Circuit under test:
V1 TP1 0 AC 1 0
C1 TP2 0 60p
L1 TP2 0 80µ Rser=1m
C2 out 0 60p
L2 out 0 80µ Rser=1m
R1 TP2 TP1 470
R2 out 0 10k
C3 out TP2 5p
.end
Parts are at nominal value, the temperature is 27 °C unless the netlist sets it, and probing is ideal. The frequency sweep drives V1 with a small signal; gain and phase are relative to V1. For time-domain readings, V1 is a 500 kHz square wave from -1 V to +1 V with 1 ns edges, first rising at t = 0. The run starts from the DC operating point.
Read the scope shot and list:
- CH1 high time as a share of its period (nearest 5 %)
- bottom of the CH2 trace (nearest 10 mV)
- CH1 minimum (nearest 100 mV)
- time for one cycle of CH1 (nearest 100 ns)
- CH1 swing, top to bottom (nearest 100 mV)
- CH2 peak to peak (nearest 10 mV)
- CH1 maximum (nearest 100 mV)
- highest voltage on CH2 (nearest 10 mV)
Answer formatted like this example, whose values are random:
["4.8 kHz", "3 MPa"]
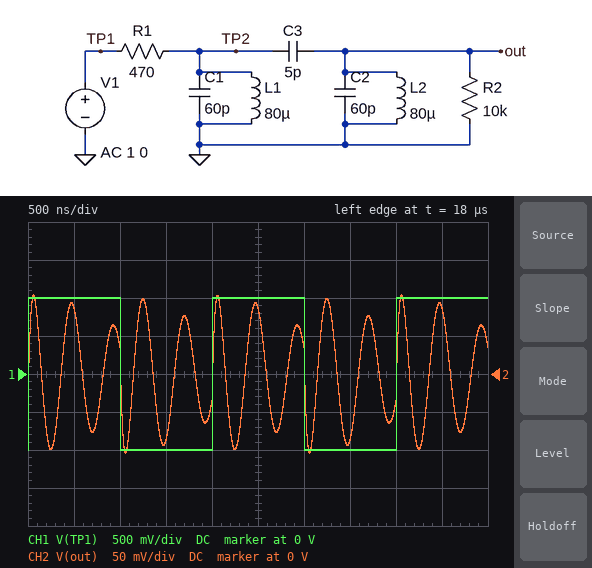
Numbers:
["50 %", "-100 mV", "-1.0 V", "2.0 µs", "2.0 V", "210 mV", "1.0 V", "100 mV"]
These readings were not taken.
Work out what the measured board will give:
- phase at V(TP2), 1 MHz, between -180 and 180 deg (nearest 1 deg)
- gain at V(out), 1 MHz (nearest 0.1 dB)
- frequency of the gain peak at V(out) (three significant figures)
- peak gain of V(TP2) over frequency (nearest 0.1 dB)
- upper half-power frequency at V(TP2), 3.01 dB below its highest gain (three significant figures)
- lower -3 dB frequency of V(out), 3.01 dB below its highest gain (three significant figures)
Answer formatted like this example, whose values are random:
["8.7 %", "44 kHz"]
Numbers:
["37 deg", "-36.0 dB", "2.21 MHz", "-0.1 dB", "6.12 MHz", "2.10 MHz"]
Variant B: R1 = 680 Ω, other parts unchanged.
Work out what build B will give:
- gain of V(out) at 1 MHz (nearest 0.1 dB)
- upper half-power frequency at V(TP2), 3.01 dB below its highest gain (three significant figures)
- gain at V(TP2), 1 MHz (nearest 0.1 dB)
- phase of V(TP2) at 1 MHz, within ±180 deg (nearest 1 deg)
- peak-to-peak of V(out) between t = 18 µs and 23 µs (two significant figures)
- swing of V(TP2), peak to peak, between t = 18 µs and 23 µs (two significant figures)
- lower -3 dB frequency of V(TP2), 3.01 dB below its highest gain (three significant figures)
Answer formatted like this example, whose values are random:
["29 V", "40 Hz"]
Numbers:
["-37.4 dB", "4.75 MHz", "-3.3 dB", "47 deg", "190 mV", "2.7 V", "1.03 MHz"]
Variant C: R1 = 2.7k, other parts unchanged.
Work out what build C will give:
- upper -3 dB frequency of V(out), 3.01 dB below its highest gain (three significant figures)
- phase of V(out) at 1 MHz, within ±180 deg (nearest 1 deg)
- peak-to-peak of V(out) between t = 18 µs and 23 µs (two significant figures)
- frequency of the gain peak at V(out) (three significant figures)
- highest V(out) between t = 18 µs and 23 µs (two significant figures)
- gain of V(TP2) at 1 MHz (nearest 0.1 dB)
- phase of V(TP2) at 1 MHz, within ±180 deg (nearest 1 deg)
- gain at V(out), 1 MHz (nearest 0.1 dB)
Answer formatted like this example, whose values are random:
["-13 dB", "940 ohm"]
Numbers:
["2.36 MHz", "-107 deg", "150 mV", "2.21 MHz", "74 mV", "-12.8 dB", "77 deg", "-46.9 dB"]
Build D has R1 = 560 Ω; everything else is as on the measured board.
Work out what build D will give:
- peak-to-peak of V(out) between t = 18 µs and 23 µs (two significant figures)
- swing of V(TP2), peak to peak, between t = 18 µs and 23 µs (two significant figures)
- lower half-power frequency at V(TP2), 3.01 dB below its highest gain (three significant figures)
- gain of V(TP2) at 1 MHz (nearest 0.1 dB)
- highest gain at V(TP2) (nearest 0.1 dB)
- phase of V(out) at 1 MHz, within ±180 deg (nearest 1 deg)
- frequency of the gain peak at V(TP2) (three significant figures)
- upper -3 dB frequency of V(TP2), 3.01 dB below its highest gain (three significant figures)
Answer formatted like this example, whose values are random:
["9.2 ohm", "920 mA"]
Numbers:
["200 mV", "2.9 V", "908 kHz", "-2.5 dB", "-0.1 dB", "-142 deg", "2.00 MHz", "5.39 MHz"]
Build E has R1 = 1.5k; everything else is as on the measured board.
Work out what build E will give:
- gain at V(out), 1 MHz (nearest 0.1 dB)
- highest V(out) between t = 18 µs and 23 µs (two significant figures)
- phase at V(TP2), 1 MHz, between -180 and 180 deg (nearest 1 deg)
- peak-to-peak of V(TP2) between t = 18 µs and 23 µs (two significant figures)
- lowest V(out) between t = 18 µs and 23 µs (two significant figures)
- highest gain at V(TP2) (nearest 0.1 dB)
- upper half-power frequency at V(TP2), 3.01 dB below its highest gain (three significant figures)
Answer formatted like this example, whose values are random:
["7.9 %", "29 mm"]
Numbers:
["-42.3 dB", "87 mV", "67 deg", "1.8 V", "-87 mV", "-0.3 dB", "3.27 MHz"]
